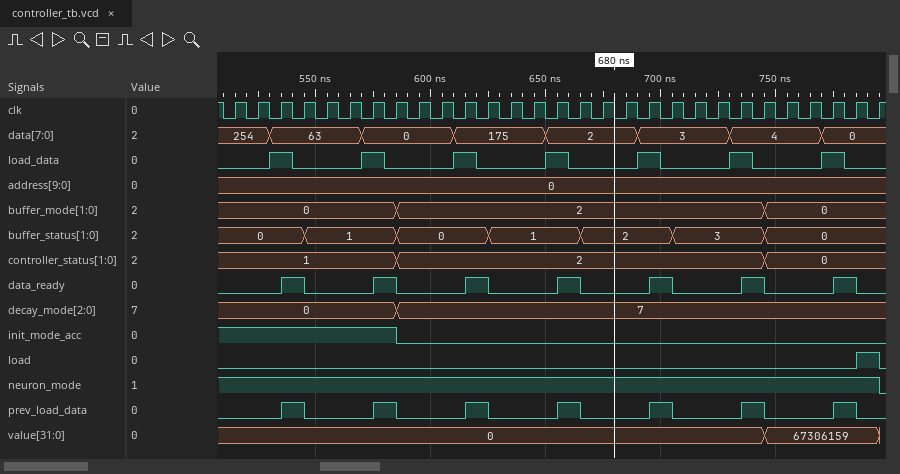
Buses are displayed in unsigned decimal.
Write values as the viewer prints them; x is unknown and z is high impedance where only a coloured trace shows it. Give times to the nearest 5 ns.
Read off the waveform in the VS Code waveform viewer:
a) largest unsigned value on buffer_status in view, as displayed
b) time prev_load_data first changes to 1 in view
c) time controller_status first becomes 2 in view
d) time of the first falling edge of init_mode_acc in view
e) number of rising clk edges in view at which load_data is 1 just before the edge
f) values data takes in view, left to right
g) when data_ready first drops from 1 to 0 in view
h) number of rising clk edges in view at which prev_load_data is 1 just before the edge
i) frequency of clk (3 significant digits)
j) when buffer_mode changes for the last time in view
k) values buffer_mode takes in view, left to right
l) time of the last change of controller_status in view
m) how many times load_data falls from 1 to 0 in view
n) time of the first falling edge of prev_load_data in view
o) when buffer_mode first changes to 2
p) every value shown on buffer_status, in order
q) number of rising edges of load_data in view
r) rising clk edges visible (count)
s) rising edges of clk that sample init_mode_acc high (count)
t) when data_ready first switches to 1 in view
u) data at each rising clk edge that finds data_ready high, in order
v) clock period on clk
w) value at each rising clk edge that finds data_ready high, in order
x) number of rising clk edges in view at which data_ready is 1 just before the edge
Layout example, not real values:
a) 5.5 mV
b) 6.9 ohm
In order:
a) 3
b) 535 ns
c) 585 ns
d) 585 ns
e) 7
f) 254, 63, 0, 175, 2, 3, 4, 0
g) 545 ns
h) 7
i) 100 MHz
j) 745 ns
k) 0, 2, 0
l) 745 ns
m) 7
n) 545 ns
o) 585 ns
p) 0, 1, 0, 1, 2, 3, 0
q) 7
r) 29
s) 8
t) 535 ns
u) 63, 0, 175, 2, 3, 4, 0
v) 10 ns
w) 0, 0, 0, 0, 0, 0, 67306159
x) 7
